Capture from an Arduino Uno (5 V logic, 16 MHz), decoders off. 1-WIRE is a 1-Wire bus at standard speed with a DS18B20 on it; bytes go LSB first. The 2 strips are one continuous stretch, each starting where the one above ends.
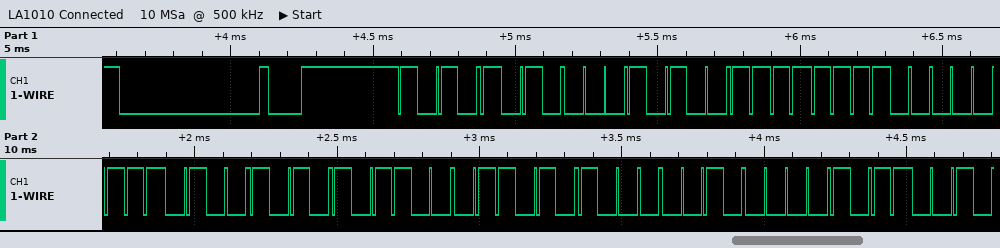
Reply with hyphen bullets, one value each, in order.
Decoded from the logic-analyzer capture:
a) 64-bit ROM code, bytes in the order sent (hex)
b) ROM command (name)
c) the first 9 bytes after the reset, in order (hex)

- 28 FF E0 52 8D 15 04 4D
- Match ROM
- 55 28 FF E0 52 8D 15 04 4D
